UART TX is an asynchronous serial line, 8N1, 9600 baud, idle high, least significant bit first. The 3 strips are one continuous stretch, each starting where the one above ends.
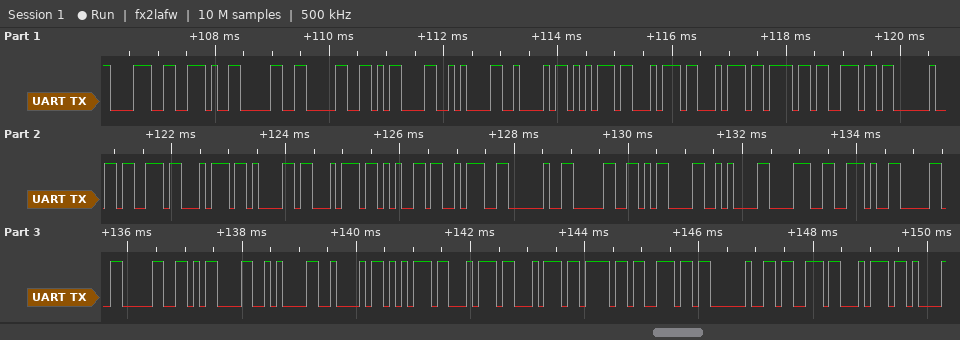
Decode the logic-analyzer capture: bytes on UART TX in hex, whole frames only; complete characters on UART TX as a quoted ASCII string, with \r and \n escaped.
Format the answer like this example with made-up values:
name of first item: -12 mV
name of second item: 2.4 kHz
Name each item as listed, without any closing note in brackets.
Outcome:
bytes on UART TX in hex, whole frames only: 38 2E 30 30 0D 0A 42 75 74 74 6F 6E 20 73 74 61 74 65 3A 20 30 0D 0A 38 2E 30 30 0D 0A 42 75 74 74 6F 6E 20 73 74
complete characters on UART TX as a quoted ASCII string, with \r and \n escaped: "8.00\r\nButton state: 0\r\n8.00\r\nButton st"
